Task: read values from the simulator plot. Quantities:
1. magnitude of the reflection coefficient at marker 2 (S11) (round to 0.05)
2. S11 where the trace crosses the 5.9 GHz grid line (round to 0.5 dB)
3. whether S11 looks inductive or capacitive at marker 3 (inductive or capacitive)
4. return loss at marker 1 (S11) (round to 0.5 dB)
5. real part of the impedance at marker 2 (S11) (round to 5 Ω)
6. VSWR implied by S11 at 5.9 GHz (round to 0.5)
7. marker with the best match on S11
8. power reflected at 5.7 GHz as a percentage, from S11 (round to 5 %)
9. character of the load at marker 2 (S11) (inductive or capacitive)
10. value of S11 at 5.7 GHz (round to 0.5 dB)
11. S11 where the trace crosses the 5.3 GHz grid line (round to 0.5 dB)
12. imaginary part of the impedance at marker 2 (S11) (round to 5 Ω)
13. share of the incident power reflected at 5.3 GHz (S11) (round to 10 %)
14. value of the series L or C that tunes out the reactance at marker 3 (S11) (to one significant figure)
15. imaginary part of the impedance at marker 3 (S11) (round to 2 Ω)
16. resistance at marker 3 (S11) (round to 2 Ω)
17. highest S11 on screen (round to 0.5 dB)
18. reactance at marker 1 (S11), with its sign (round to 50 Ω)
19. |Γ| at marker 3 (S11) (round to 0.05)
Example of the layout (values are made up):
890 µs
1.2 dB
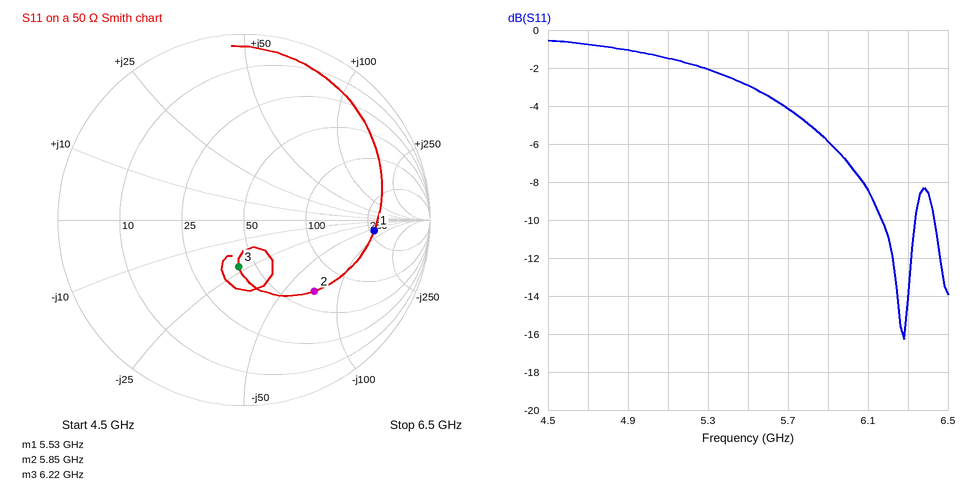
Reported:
0.55
-6.0 dB
capacitive
3.0 dB
65 Ω
3.0
marker 3
40 %
capacitive
-4.0 dB
-2.0 dB
-70 Ω
60 %
600 pH
-22 Ω
42 Ω
-0.5 dB
-50 Ω
0.25
